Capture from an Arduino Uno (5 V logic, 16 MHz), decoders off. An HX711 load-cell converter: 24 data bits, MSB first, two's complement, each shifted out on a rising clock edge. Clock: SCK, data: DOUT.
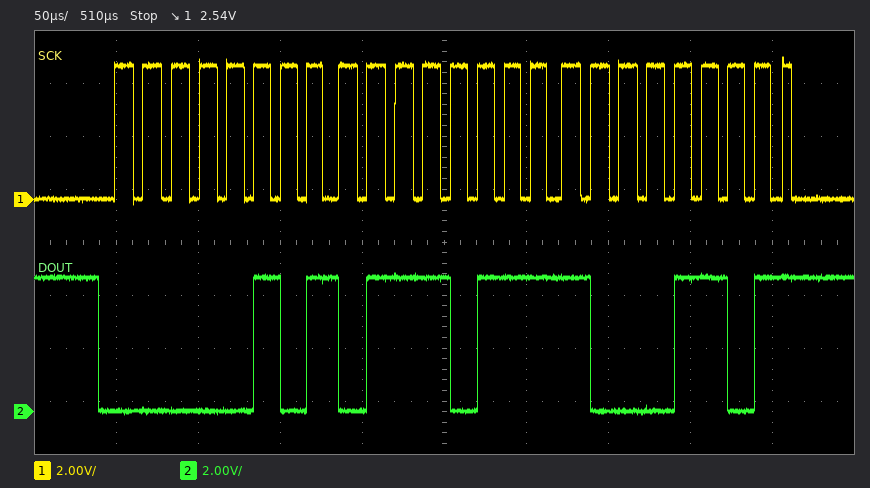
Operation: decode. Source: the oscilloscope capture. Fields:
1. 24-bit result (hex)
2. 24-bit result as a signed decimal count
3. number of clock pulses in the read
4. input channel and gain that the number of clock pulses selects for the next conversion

0x05778D
358285
25
channel A, gain 128
